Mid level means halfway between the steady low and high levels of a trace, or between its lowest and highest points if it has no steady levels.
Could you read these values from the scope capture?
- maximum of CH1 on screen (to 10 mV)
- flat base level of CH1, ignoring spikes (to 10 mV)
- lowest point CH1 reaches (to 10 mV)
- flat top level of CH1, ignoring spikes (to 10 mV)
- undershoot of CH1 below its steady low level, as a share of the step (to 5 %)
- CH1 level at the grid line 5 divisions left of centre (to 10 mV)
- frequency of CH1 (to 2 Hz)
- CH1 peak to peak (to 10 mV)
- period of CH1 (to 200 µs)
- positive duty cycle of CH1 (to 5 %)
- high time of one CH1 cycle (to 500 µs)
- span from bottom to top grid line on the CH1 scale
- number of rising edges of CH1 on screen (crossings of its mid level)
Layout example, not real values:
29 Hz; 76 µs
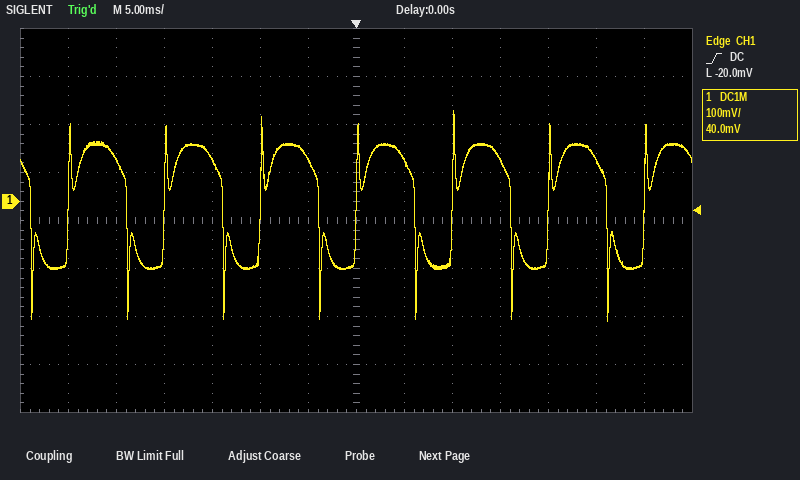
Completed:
190 mV; -140 mV; -250 mV; 120 mV; 45 %; 90 mV; 100 Hz; 440 mV; 10.0 ms; 60 %; 6.0 ms; 800 mV; 7
